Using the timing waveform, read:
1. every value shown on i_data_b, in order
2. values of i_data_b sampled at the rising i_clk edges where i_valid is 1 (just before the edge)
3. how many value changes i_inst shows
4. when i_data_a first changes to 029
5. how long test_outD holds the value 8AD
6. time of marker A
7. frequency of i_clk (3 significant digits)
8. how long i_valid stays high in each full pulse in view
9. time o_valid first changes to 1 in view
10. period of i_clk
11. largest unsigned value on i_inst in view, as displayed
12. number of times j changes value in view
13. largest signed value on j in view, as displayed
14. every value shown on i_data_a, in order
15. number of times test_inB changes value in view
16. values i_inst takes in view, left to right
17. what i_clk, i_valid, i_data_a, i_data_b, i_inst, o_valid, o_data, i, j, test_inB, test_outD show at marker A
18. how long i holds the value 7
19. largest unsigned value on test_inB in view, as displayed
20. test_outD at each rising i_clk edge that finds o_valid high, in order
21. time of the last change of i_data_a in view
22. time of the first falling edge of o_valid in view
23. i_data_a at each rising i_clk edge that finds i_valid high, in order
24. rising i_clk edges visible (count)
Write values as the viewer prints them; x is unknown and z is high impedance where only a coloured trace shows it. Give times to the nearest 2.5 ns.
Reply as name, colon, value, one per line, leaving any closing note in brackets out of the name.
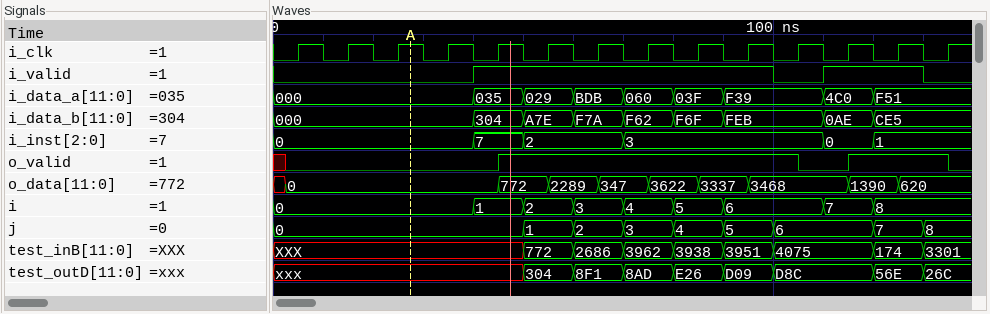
every value shown on i_data_b, in order: 000, 304, A7E, F7A, F62, F6F, FEB, 0AE, CE5
values of i_data_b sampled at the rising i_clk edges where i_valid is 1: 304, A7E, F7A, F62, F6F, FEB, 0AE, CE5
how many value changes i_inst shows: 5
when i_data_a first changes to 029: 50 ns
how long test_outD holds the value 8AD: 10 ns
time of marker A: 27.5 ns
frequency of i_clk: 100 MHz
how long i_valid stays high in each full pulse in view: 60 ns, 20 ns
time o_valid first changes to 1 in view: 45 ns
period of i_clk: 10 ns
largest unsigned value on i_inst in view, as displayed: 7
number of times j changes value in view: 8
largest signed value on j in view, as displayed: 8
every value shown on i_data_a, in order: 000, 035, 029, BDB, 060, 03F, F39, 4C0, F51
number of times test_inB changes value in view: 8
values i_inst takes in view, left to right: 0, 7, 2, 3, 0, 1
what i_clk, i_valid, i_data_a, i_data_b, i_inst, o_valid, o_data, i, j, test_inB, test_outD show at marker A: i_clk=1, i_valid=0, i_data_a=000, i_data_b=000, i_inst=0, o_valid=0, o_data=0, i=0, j=0, test_inB=XXX, test_outD=xxx
how long i holds the value 7: 10 ns
largest unsigned value on test_inB in view, as displayed: 4075
test_outD at each rising i_clk edge that finds o_valid high, in order: 304, 8F1, 8AD, E26, D09, D8C, 56E, 26C
time of the last change of i_data_a in view: 120 ns
time of the first falling edge of o_valid in view: 105 ns
i_data_a at each rising i_clk edge that finds i_valid high, in order: 035, 029, BDB, 060, 03F, F39, 4C0, F51
rising i_clk edges visible: 14
